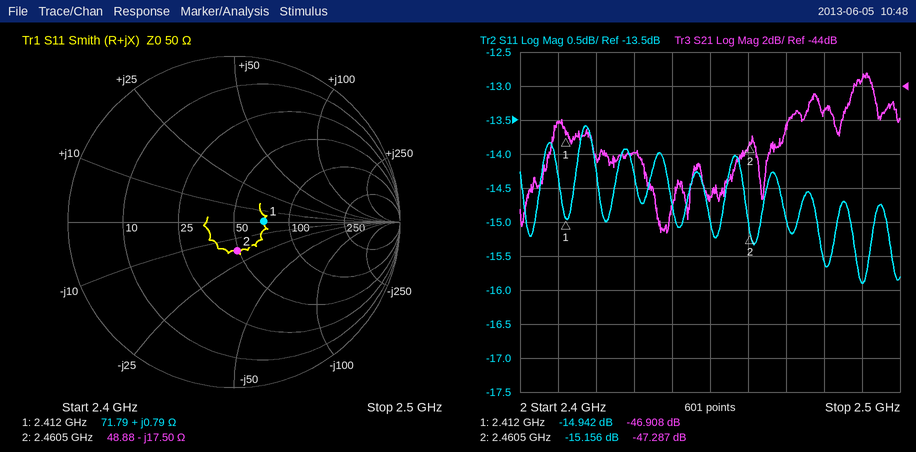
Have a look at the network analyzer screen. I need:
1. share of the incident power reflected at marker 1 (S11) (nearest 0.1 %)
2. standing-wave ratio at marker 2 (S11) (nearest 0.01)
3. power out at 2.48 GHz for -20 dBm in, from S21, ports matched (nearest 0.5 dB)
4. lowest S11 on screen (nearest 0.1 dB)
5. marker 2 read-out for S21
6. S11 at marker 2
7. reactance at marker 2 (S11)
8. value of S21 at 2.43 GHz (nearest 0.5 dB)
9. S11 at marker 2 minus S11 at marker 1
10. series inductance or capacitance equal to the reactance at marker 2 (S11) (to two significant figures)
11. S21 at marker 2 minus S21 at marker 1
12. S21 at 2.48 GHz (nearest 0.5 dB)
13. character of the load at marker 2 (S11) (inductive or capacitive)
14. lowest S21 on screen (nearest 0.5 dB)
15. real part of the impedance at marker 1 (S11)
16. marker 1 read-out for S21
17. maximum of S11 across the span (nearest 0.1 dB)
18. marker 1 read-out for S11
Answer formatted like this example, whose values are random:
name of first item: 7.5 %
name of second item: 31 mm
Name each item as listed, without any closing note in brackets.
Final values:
share of the incident power reflected at marker 1 (S11): 3.2 %
standing-wave ratio at marker 2 (S11): 1.42
power out at 2.48 GHz for -20 dBm in, from S21, ports matched: -65.5 dBm
lowest S11 on screen: -15.9 dB
marker 2 read-out for S21: -47.287 dB
S11 at marker 2: -15.156 dB
reactance at marker 2: -17.50 Ω
value of S21 at 2.43 GHz: -48.0 dB
S11 at marker 2 minus S11 at marker 1: -0.214 dB
series inductance or capacitance equal to the reactance at marker 2 (S11): 3.7 pF
S21 at marker 2 minus S21 at marker 1: -0.379 dB
S21 at 2.48 GHz: -45.5 dB
character of the load at marker 2 (S11): capacitive
lowest S21 on screen: -52.5 dB
real part of the impedance at marker 1: 71.79 Ω
marker 1 read-out for S21: -46.908 dB
maximum of S11 across the span: -13.6 dB
marker 1 read-out for S11: -14.942 dB
